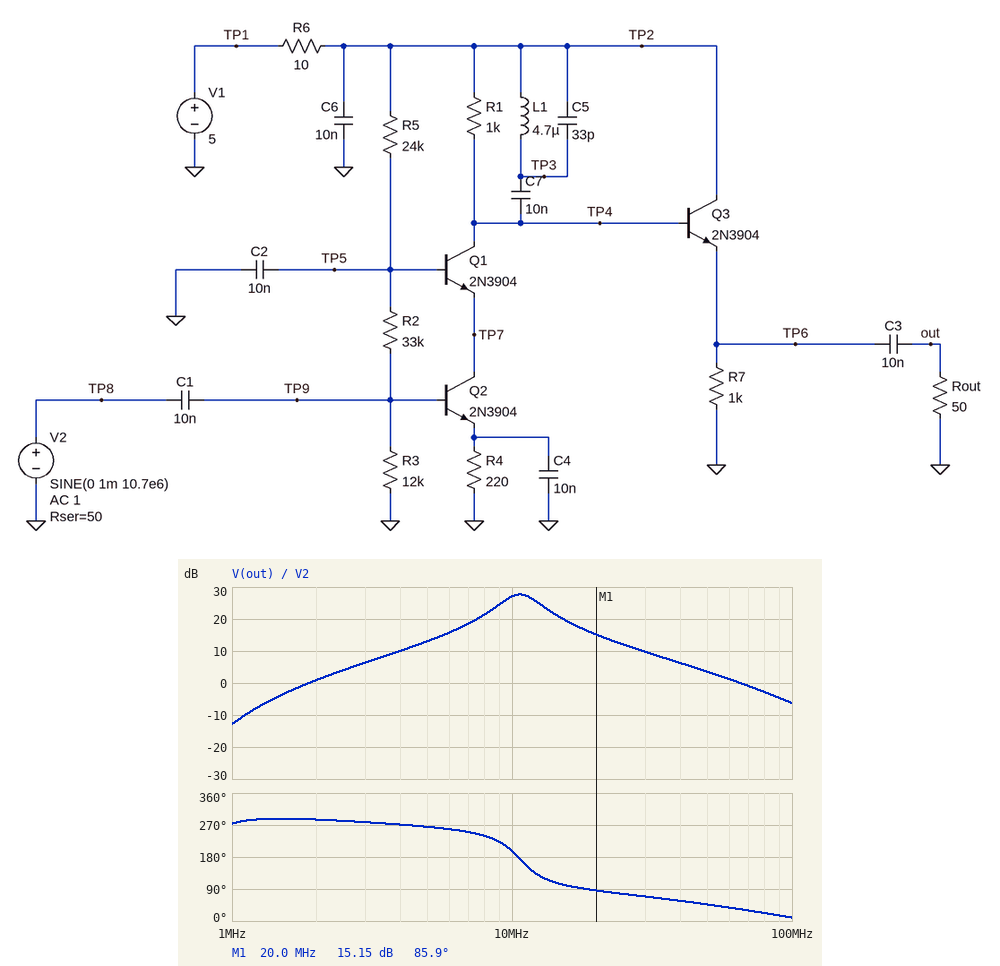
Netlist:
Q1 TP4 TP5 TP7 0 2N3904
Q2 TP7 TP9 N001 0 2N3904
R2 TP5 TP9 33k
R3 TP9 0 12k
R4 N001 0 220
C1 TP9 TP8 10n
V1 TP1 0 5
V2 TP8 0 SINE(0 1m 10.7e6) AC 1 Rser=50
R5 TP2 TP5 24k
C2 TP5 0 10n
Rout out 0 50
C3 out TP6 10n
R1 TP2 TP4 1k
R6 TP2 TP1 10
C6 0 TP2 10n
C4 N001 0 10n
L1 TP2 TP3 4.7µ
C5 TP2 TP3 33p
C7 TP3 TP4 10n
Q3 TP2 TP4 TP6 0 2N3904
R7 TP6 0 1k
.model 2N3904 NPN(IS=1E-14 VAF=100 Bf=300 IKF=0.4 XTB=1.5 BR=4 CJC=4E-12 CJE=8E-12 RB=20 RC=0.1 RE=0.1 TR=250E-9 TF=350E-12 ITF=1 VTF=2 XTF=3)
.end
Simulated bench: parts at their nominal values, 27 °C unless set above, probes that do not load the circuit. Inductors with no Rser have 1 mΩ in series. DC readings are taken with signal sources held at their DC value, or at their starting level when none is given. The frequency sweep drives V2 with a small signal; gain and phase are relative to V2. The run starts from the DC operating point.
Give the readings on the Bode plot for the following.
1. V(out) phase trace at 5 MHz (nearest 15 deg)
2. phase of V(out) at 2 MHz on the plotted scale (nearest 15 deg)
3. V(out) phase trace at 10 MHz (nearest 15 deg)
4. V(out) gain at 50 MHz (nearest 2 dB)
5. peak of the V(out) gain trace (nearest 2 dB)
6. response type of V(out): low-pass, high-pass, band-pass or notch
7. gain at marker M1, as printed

270 deg
285 deg
195 deg
4 dB
28 dB
band-pass
15.15 dB
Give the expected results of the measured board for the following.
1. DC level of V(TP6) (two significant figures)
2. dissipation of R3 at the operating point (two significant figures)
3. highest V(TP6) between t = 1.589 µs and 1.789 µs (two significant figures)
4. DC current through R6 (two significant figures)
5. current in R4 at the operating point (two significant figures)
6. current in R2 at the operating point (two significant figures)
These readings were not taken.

3.5 V
57 µW
3.5 V
4.3 mA
800 µA
71 µA
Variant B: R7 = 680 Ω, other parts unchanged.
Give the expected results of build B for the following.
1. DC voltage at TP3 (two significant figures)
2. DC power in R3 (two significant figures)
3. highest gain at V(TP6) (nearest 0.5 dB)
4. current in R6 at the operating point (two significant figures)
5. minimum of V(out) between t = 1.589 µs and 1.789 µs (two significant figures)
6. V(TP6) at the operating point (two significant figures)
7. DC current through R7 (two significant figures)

4.9 V
56 µW
28.0 dB
5.9 mA
-25 mV
3.4 V
5.1 mA
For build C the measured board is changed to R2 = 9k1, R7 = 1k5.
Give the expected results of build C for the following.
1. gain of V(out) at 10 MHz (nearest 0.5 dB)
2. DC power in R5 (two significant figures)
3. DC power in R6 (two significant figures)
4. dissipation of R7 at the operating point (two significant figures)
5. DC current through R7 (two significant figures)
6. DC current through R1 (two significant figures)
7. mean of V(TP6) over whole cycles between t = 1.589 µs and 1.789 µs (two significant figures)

34.5 dB
320 µW
140 µW
2.5 mW
1.3 mA
2.4 mA
1.9 V
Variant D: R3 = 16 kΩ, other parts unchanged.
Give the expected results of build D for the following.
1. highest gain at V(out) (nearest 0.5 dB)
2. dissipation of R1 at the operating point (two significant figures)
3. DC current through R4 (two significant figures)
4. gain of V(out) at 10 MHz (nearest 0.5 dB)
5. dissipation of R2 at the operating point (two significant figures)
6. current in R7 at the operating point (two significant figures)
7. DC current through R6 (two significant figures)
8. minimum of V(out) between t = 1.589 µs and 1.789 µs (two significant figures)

33.0 dB
2.3 mW
1.5 mA
32.5 dB
150 µW
2.8 mA
4.3 mA
-43 mV
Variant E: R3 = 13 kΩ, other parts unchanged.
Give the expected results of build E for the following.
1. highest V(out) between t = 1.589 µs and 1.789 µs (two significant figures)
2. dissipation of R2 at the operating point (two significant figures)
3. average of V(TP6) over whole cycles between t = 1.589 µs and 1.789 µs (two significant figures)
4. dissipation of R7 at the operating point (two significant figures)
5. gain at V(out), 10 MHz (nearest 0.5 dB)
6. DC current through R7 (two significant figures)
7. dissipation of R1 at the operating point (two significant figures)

30 mV
160 µW
3.3 V
11 mW
29.0 dB
3.3 mA
980 µW
